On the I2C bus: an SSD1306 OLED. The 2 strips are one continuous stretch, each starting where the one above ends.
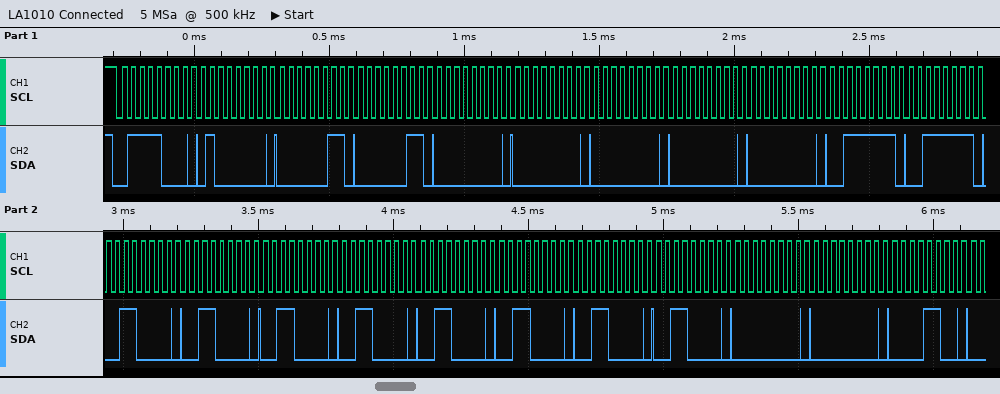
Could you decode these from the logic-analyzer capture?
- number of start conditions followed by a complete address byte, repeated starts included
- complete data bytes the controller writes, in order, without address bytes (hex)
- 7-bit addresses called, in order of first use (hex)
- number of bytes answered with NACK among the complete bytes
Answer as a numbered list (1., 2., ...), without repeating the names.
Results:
1. 1
2. 40 03 03 00 00 00 00 00 3F 3F 30 30 30 30 30 30 30 30 00 00 0C
3. 0x3C
4. 0
